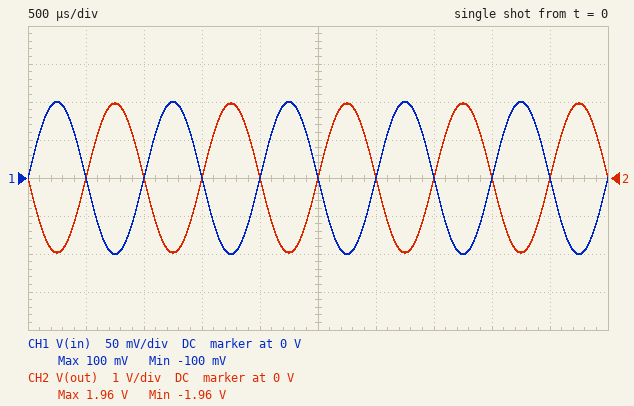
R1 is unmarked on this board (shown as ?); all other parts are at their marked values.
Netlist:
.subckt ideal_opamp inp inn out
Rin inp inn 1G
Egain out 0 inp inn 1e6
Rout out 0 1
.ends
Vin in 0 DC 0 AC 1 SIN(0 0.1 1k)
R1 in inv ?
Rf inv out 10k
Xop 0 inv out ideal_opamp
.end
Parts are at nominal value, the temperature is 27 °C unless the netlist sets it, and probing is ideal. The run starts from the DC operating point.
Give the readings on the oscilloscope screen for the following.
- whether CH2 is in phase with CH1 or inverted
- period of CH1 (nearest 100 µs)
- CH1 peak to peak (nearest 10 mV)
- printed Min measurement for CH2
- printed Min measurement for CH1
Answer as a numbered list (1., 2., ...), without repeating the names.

1. inverted
2. 1.0 ms
3. 200 mV
4. -1.96 V
5. -100 mV
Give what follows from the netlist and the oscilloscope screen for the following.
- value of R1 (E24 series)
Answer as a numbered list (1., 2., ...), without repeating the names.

1. 510 Ω
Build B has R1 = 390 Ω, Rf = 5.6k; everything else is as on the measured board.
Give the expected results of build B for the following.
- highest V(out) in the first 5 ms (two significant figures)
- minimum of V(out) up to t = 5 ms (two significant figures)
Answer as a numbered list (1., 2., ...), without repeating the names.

1. 1.4 V
2. -1.4 V
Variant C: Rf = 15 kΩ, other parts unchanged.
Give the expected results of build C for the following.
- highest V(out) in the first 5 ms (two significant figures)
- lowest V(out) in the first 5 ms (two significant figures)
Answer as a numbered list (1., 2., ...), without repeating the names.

1. 2.9 V
2. -2.9 V
